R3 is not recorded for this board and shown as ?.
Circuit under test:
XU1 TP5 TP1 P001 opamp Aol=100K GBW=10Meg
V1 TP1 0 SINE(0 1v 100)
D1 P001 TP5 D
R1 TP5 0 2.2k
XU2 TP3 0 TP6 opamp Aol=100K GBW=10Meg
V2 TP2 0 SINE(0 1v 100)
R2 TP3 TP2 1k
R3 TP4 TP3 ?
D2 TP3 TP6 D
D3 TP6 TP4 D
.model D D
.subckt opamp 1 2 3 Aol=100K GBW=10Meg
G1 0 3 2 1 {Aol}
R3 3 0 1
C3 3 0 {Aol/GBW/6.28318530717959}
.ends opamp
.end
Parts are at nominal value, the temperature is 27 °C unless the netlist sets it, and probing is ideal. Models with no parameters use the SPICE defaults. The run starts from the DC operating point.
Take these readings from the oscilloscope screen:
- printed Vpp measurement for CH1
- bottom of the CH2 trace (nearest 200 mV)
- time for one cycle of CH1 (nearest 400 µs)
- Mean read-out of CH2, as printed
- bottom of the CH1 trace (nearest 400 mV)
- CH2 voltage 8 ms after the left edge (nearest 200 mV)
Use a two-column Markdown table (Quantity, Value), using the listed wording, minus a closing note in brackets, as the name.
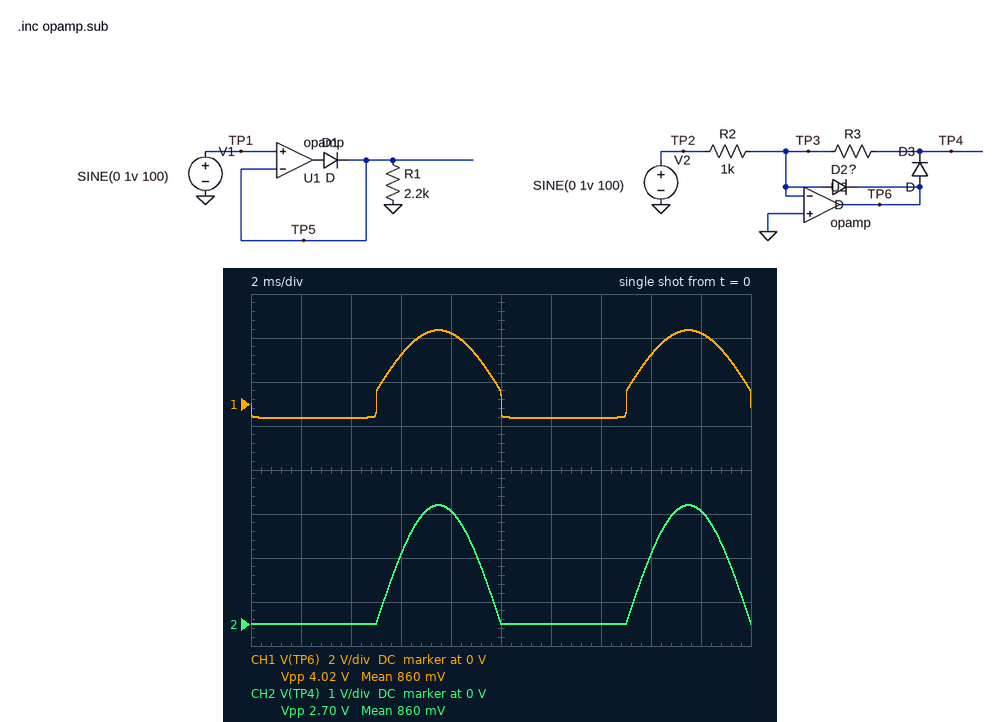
| Quantity | Value |
|---|---|
| printed Vpp measurement for CH1 | 4.02 V |
| bottom of the CH2 trace | 0 V |
| time for one cycle of CH1 | 10.0 ms |
| Mean read-out of CH2, as printed | 860 mV |
| bottom of the CH1 trace | -800 mV |
| CH2 voltage 8 ms after the left edge | 2.6 V |
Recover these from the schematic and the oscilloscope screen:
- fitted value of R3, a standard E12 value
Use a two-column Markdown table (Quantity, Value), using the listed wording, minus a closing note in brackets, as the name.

| Quantity | Value |
|---|---|
| fitted value of R3, a standard E12 value | 2.7 kΩ |
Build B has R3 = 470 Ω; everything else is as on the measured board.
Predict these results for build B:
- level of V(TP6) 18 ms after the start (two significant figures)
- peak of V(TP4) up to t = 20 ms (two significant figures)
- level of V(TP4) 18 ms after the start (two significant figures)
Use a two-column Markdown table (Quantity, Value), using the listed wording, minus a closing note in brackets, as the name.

| Quantity | Value |
|---|---|
| level of V(TP6) 18 ms after the start | 1.1 V |
| peak of V(TP4) up to t = 20 ms | 470 mV |
| level of V(TP4) 18 ms after the start | 450 mV |
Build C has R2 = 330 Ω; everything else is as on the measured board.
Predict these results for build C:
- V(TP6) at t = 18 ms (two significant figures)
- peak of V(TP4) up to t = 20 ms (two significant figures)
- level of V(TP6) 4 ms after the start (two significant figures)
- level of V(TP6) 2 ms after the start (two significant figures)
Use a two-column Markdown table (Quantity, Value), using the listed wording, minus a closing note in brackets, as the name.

| Quantity | Value |
|---|---|
| V(TP6) at t = 18 ms | 8.5 V |
| peak of V(TP4) up to t = 20 ms | 8.2 V |
| level of V(TP6) 4 ms after the start | -670 mV |
| level of V(TP6) 2 ms after the start | -680 mV |
